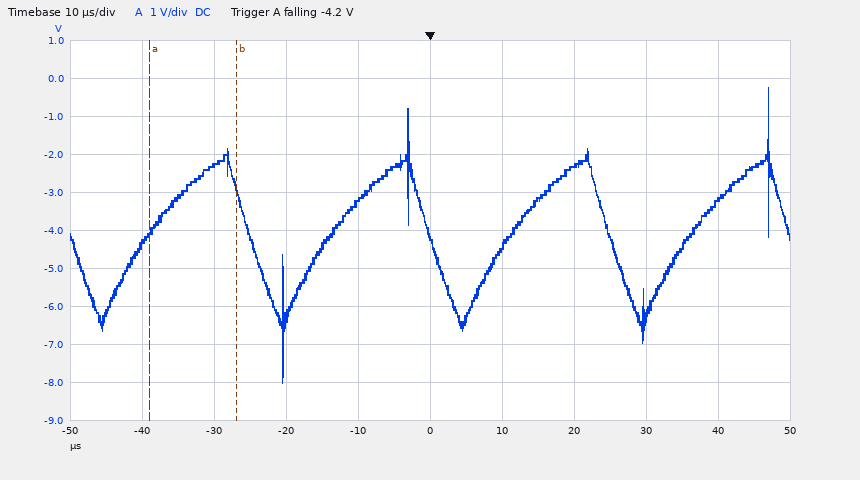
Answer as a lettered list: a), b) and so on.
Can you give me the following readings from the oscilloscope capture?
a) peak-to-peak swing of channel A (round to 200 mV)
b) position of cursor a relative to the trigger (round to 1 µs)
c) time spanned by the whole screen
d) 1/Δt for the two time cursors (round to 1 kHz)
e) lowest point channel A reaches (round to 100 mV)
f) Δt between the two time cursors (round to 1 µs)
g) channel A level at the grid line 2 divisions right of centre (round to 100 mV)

a) 7.8 V
b) -39 µs
c) 100 µs
d) 83 kHz
e) -8.0 V
f) 12 µs
g) -2.3 V
